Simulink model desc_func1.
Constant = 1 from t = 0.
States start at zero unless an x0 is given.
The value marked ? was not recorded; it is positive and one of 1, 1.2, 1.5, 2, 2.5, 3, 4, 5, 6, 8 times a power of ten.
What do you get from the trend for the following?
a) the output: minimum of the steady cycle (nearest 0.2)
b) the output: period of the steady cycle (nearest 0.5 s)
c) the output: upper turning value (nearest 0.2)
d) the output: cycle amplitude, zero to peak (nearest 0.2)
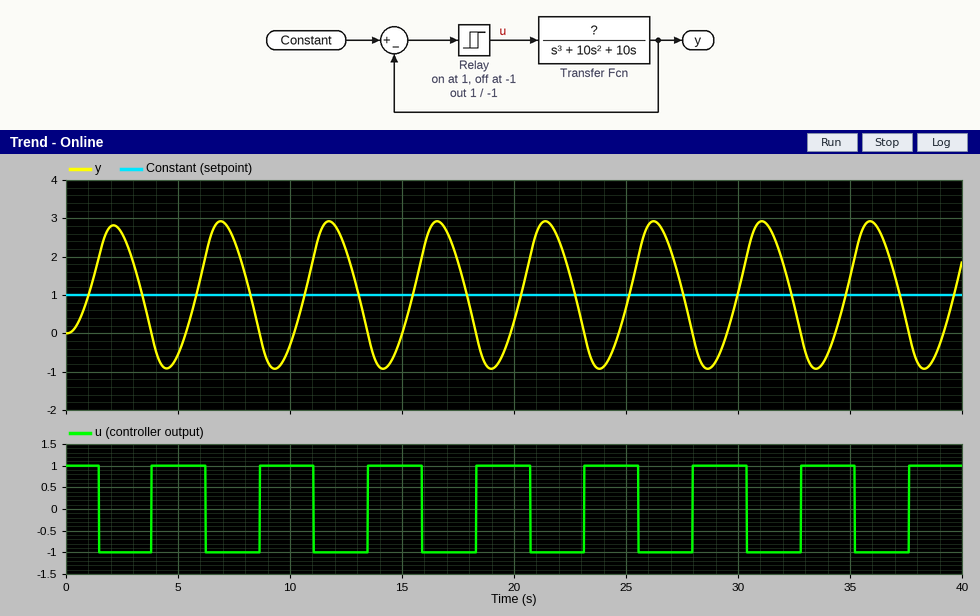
-1.0
5.0 s
3.0
2.0
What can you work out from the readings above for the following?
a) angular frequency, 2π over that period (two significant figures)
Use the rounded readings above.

1.3 rad/s
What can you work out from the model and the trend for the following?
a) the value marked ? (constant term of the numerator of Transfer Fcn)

30
